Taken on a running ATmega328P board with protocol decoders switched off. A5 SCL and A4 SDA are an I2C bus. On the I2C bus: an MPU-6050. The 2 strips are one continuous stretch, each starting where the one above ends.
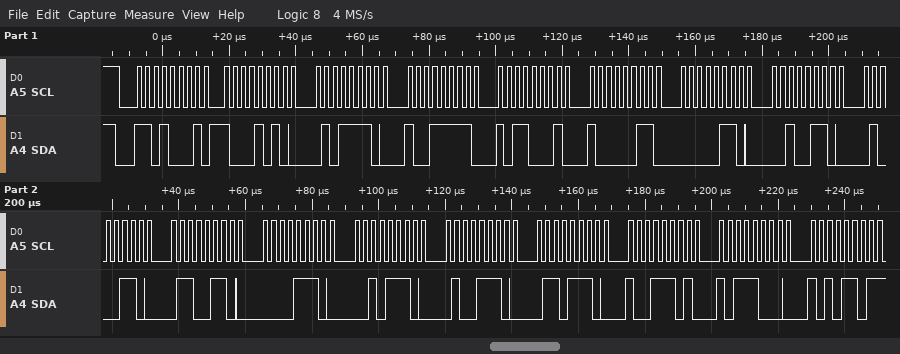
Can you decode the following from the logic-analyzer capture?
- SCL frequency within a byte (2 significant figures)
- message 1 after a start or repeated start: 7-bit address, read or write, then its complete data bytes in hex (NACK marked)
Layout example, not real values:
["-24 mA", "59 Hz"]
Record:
["400 kHz", "0x68 read: 8A 5E 9F B1 83 06 26 46 66 0E 2E 4E 6E 9D B8 AD NACK"]
